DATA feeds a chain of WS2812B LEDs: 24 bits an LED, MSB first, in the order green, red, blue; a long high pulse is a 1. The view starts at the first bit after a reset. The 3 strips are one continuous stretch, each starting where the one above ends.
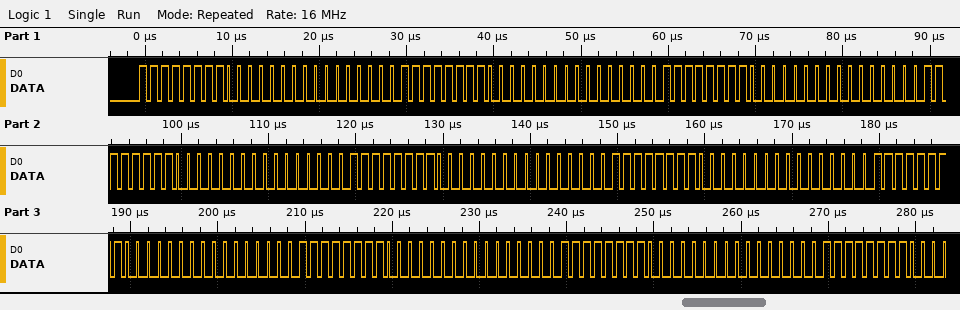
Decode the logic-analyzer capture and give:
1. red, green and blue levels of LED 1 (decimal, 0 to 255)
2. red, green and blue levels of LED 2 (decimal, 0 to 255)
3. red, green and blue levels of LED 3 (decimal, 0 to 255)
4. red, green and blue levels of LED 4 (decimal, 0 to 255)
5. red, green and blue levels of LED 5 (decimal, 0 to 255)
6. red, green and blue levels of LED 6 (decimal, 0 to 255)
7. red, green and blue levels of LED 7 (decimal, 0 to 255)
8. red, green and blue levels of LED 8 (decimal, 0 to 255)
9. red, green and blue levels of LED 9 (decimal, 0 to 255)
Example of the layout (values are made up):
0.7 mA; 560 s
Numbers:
0, 255, 0; 0, 255, 0; 0, 255, 0; 0, 255, 0; 0, 255, 0; 0, 255, 0; 0, 255, 0; 0, 255, 0; 0, 255, 0
